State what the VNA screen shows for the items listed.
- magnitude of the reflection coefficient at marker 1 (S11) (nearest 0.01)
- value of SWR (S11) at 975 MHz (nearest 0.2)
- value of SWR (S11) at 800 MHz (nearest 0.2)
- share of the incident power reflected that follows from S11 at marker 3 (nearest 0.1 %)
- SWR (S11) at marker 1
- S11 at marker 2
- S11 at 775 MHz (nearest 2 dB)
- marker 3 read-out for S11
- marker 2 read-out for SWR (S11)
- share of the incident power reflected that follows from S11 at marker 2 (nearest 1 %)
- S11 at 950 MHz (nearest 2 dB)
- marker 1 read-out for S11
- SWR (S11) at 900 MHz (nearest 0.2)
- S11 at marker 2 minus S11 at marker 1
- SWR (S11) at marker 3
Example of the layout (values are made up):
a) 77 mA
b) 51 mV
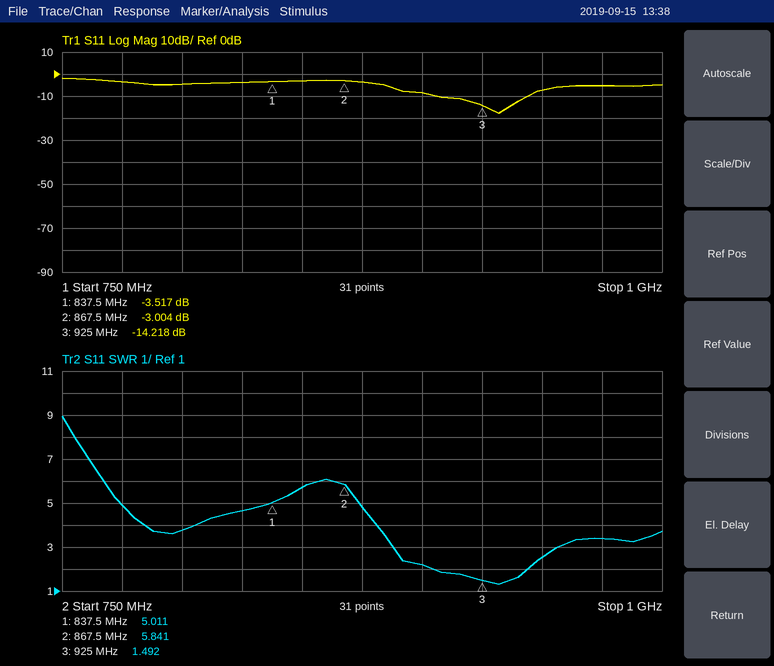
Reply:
a) 0.67
b) 3.4
c) 3.8
d) 3.8 %
e) 5.011
f) -3.004 dB
g) -4 dB
h) -14.218 dB
i) 5.841
j) 50 %
k) -8 dB
l) -3.517 dB
m) 2.2
n) 0.513 dB
o) 1.492
